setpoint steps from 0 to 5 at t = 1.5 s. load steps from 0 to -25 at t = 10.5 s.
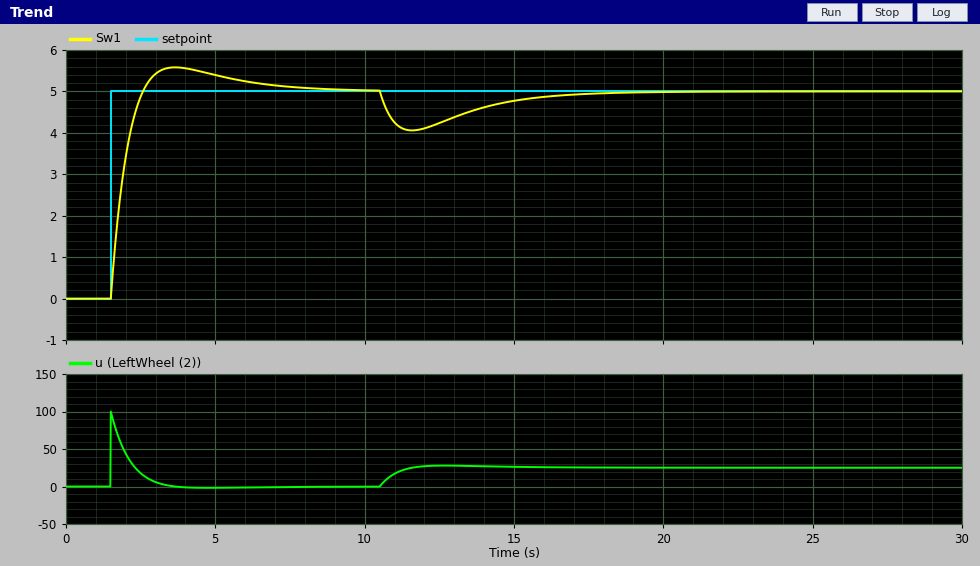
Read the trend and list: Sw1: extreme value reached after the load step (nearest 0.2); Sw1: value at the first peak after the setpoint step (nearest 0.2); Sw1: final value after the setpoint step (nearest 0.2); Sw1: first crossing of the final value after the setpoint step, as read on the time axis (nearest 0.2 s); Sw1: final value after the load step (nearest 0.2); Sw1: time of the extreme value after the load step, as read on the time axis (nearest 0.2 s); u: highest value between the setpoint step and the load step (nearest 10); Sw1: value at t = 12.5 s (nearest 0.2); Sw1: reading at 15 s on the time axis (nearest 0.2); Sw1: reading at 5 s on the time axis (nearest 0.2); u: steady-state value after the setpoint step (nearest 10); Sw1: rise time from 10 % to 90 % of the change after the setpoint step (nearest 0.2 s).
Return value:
4.0
5.6
5.0
2.6 s
5.0
11.6 s
100
4.2
4.8
5.4
0
0.8 s
